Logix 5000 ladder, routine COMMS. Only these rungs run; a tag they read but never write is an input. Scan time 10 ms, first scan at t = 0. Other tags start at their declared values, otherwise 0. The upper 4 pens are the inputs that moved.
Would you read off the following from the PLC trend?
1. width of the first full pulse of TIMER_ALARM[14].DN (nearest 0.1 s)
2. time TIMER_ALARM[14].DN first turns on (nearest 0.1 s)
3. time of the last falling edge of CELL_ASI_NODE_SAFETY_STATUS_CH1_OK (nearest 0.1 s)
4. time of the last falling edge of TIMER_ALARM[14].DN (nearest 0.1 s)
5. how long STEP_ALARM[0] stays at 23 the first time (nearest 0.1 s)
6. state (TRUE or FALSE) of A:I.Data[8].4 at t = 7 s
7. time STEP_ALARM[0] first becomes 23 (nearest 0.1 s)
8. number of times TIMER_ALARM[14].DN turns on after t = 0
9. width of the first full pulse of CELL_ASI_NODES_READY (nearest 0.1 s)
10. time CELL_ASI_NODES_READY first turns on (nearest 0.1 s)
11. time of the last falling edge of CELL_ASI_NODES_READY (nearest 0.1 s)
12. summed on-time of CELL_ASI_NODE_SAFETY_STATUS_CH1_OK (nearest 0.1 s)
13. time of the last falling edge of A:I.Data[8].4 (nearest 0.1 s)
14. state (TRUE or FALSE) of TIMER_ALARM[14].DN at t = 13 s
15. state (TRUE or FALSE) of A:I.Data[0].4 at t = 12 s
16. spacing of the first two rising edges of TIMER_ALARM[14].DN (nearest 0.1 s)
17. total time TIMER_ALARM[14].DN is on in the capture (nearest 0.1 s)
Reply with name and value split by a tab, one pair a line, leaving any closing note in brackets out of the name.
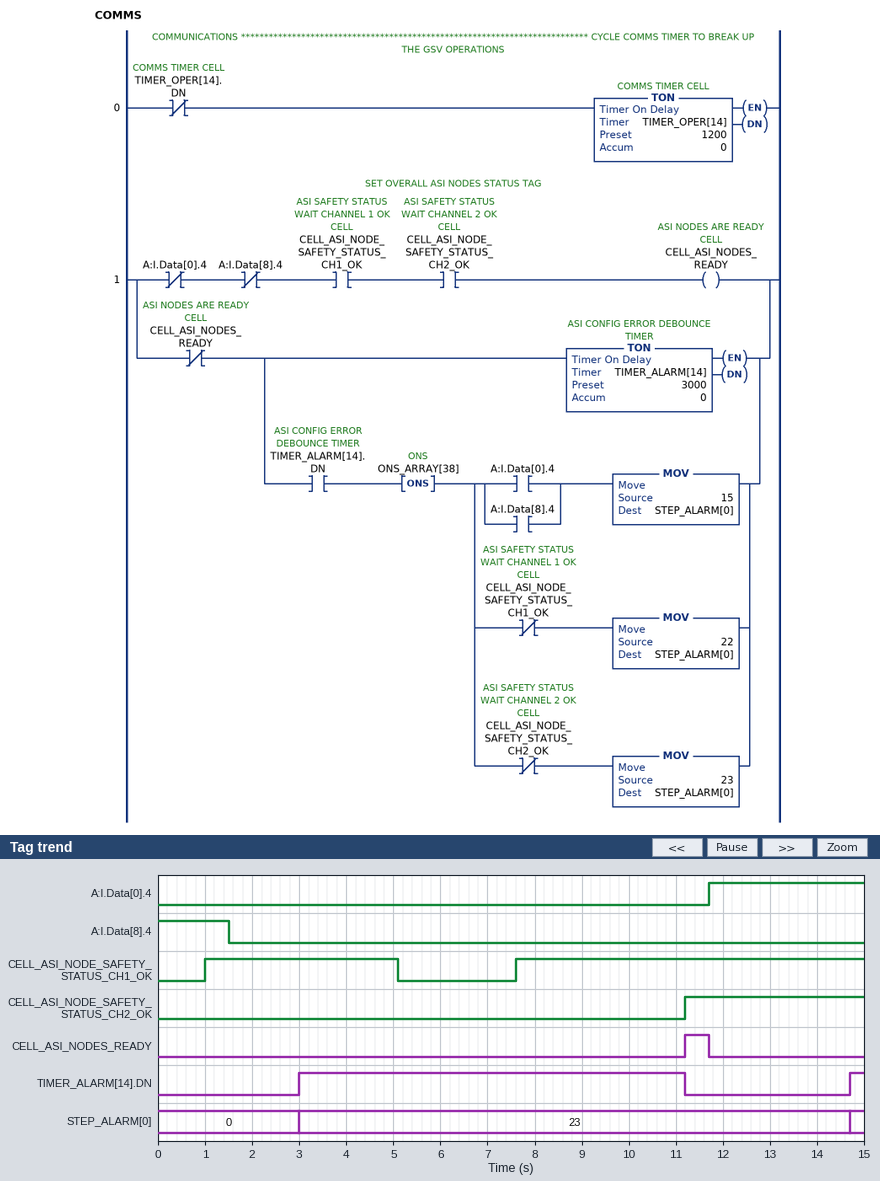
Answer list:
width of the first full pulse of TIMER_ALARM[14].DN	8.2 s
time TIMER_ALARM[14].DN first turns on	3.0 s
time of the last falling edge of CELL_ASI_NODE_SAFETY_STATUS_CH1_OK	5.1 s
time of the last falling edge of TIMER_ALARM[14].DN	11.2 s
how long STEP_ALARM[0] stays at 23 the first time	11.7 s
state (TRUE or FALSE) of A:I.Data[8].4 at t = 7 s	FALSE
time STEP_ALARM[0] first becomes 23	3.0 s
number of times TIMER_ALARM[14].DN turns on after t = 0	2
width of the first full pulse of CELL_ASI_NODES_READY	0.5 s
time CELL_ASI_NODES_READY first turns on	11.2 s
time of the last falling edge of CELL_ASI_NODES_READY	11.7 s
summed on-time of CELL_ASI_NODE_SAFETY_STATUS_CH1_OK	11.5 s
time of the last falling edge of A:I.Data[8].4	1.5 s
state (TRUE or FALSE) of TIMER_ALARM[14].DN at t = 13 s	FALSE
state (TRUE or FALSE) of A:I.Data[0].4 at t = 12 s	TRUE
spacing of the first two rising edges of TIMER_ALARM[14].DN	11.7 s
total time TIMER_ALARM[14].DN is on in the capture	8.5 s
